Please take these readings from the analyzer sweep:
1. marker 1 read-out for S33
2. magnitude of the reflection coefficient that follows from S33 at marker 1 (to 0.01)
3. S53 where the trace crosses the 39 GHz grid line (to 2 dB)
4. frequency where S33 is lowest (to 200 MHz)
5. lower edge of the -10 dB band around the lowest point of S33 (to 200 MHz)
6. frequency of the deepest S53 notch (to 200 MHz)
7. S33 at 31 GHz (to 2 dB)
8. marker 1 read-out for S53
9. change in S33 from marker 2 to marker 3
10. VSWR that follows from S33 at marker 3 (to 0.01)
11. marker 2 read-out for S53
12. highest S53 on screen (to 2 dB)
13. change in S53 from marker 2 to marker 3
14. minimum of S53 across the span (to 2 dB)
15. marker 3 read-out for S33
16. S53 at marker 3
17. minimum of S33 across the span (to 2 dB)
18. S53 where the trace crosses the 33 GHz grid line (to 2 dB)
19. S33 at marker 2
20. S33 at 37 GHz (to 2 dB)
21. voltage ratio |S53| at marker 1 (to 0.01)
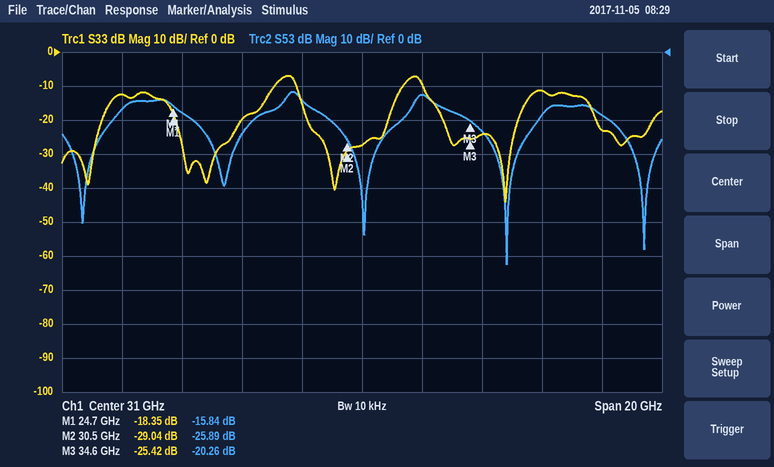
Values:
-18.35 dB
0.12
-18 dB
35.8 GHz
33.0 GHz
35.8 GHz
-28 dB
-15.84 dB
3.62 dB
1.11
-25.89 dB
-12 dB
5.63 dB
-62 dB
-25.42 dB
-20.26 dB
-44 dB
-12 dB
-29.04 dB
-12 dB
0.16
